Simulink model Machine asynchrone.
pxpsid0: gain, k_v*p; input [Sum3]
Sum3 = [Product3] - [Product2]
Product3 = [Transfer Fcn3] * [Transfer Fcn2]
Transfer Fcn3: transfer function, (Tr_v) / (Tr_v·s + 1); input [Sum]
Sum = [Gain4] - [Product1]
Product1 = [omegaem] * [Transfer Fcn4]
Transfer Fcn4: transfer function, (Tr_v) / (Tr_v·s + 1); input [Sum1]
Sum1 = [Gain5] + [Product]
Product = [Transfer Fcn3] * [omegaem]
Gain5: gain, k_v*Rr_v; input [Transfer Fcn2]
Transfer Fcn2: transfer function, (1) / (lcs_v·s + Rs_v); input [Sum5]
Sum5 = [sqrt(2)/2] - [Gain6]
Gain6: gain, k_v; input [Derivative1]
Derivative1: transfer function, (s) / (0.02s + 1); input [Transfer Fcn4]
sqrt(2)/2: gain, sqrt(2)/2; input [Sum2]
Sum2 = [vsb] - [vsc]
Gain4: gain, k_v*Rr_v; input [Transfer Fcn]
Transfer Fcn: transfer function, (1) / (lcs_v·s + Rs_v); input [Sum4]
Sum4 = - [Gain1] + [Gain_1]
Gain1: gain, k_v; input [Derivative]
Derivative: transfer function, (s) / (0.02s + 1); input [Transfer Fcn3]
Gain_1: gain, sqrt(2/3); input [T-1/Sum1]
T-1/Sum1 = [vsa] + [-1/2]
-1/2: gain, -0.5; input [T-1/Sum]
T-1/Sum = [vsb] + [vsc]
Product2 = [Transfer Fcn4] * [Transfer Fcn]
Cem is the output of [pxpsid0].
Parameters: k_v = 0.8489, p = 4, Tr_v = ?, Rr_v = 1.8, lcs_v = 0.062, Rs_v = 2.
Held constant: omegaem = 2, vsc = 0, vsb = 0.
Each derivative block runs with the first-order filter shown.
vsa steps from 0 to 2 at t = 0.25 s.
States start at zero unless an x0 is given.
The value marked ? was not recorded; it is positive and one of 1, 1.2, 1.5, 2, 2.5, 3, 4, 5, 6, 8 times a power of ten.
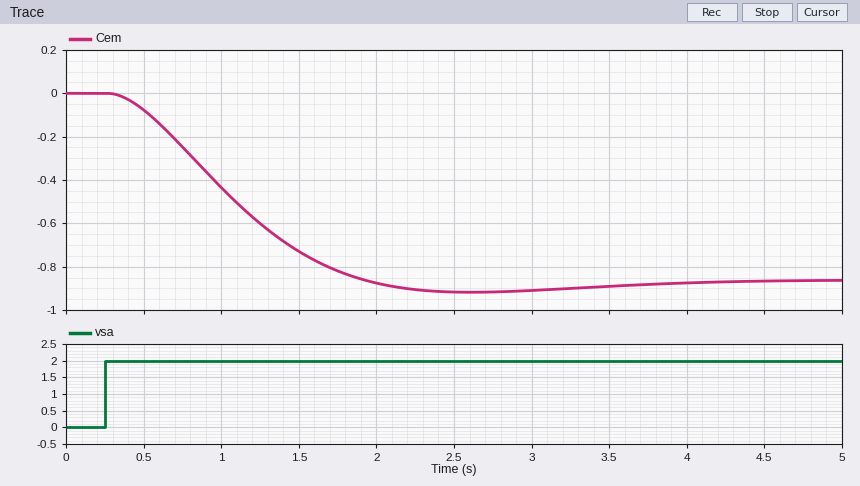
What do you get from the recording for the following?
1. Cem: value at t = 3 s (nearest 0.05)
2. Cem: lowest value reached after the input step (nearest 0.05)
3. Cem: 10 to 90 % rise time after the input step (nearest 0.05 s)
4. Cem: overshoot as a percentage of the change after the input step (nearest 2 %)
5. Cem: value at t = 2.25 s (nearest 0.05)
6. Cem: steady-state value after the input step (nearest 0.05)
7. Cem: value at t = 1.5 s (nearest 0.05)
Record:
-0.90
-0.90
1.10 s
6 %
-0.90
-0.85
-0.75
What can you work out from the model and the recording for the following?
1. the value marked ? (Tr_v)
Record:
0.5
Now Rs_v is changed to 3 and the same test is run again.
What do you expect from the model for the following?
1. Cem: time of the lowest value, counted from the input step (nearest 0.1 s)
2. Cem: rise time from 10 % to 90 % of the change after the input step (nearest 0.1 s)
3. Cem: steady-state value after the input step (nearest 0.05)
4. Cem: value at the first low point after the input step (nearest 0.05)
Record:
2.1 s
1.0 s
-0.40
-0.40
